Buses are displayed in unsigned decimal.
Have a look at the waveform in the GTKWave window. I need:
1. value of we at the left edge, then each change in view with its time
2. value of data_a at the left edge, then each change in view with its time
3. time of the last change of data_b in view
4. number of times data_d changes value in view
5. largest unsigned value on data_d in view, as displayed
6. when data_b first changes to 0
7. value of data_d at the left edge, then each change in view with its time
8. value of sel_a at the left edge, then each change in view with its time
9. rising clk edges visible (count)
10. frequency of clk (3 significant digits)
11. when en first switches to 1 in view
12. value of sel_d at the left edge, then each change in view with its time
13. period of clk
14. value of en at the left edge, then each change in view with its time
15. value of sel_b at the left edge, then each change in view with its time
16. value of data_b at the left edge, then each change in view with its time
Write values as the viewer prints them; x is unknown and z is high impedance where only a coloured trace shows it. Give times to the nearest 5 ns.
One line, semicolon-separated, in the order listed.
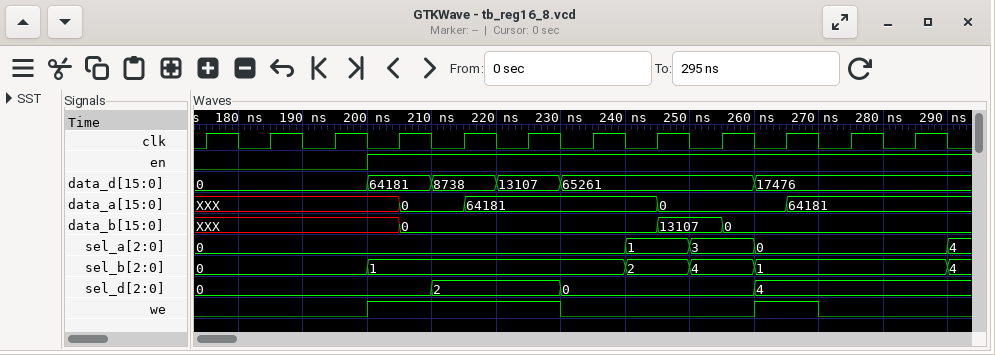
0, 1 at 200 ns, 0 at 230 ns, 1 at 260 ns, 0 at 270 ns; XXX, 0 at 205 ns, 64181 at 215 ns, 0 at 245 ns, 64181 at 265 ns; 255 ns; 5; 65261; 205 ns; 0, 64181 at 200 ns, 8738 at 210 ns, 13107 at 220 ns, 65261 at 230 ns, 17476 at 260 ns; 0, 1 at 240 ns, 3 at 250 ns, 0 at 260 ns, 4 at 290 ns; 12; 100 MHz; 200 ns; 0, 2 at 210 ns, 0 at 230 ns, 4 at 260 ns; 10 ns; 0, 1 at 200 ns; 0, 1 at 200 ns, 2 at 240 ns, 4 at 250 ns, 1 at 260 ns, 4 at 290 ns; XXX, 0 at 205 ns, 13107 at 245 ns, 0 at 255 ns
